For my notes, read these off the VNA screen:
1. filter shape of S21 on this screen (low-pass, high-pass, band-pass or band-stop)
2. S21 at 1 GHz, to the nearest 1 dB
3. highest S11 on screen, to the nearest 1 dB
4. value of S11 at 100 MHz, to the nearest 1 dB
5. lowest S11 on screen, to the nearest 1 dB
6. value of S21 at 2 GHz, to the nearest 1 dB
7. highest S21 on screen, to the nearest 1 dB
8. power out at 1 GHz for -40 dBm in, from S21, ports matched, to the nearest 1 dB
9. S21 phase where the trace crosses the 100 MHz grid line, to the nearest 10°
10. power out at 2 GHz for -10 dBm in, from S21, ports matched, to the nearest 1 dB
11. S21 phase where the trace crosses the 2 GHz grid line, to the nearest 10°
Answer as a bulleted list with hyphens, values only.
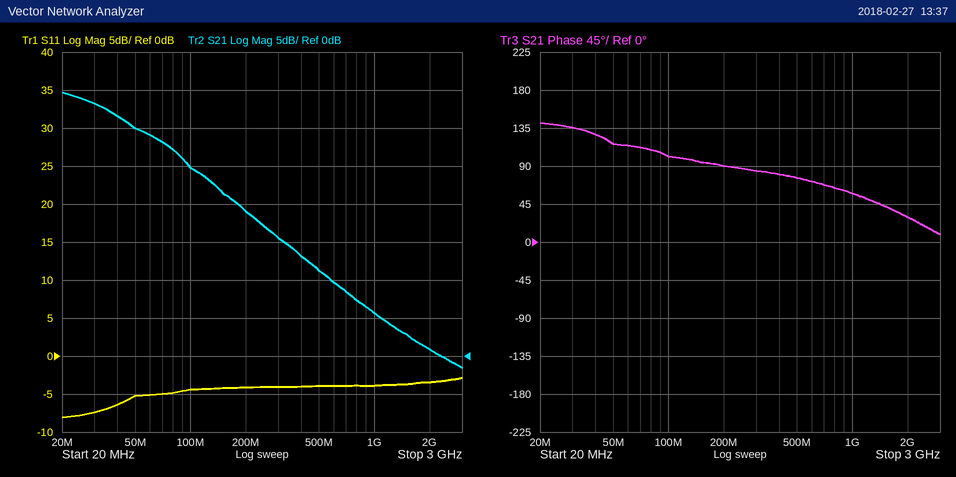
- low-pass
- 6 dB
- -3 dB
- -4 dB
- -8 dB
- 1 dB
- 35 dB
- -34 dBm
- 100°
- -9 dBm
- 30°
